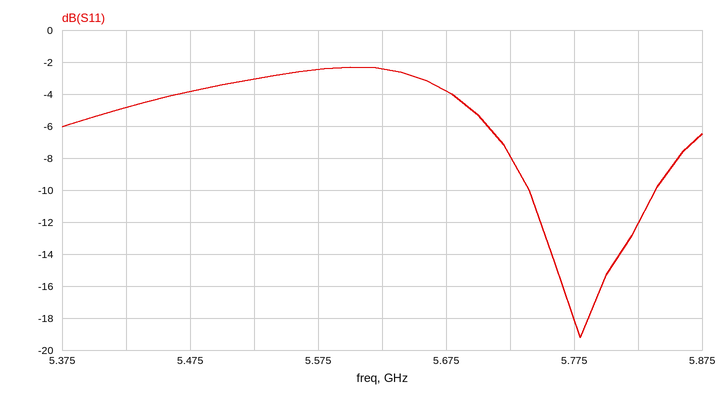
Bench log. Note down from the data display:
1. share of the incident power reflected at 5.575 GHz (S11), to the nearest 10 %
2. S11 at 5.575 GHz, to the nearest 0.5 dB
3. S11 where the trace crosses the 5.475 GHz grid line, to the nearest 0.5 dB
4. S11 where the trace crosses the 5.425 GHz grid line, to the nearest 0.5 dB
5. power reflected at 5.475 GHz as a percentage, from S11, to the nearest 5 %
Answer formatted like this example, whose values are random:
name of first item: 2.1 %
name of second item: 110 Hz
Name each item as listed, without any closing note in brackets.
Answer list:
share of the incident power reflected at 5.575 GHz (S11), to the nearest 10 %: 60 %
S11 at 5.575 GHz, to the nearest 0.5 dB: -2.5 dB
S11 where the trace crosses the 5.475 GHz grid line, to the nearest 0.5 dB: -4.0 dB
S11 where the trace crosses the 5.425 GHz grid line, to the nearest 0.5 dB: -5.0 dB
power reflected at 5.475 GHz as a percentage, from S11, to the nearest 5 %: 40 %
